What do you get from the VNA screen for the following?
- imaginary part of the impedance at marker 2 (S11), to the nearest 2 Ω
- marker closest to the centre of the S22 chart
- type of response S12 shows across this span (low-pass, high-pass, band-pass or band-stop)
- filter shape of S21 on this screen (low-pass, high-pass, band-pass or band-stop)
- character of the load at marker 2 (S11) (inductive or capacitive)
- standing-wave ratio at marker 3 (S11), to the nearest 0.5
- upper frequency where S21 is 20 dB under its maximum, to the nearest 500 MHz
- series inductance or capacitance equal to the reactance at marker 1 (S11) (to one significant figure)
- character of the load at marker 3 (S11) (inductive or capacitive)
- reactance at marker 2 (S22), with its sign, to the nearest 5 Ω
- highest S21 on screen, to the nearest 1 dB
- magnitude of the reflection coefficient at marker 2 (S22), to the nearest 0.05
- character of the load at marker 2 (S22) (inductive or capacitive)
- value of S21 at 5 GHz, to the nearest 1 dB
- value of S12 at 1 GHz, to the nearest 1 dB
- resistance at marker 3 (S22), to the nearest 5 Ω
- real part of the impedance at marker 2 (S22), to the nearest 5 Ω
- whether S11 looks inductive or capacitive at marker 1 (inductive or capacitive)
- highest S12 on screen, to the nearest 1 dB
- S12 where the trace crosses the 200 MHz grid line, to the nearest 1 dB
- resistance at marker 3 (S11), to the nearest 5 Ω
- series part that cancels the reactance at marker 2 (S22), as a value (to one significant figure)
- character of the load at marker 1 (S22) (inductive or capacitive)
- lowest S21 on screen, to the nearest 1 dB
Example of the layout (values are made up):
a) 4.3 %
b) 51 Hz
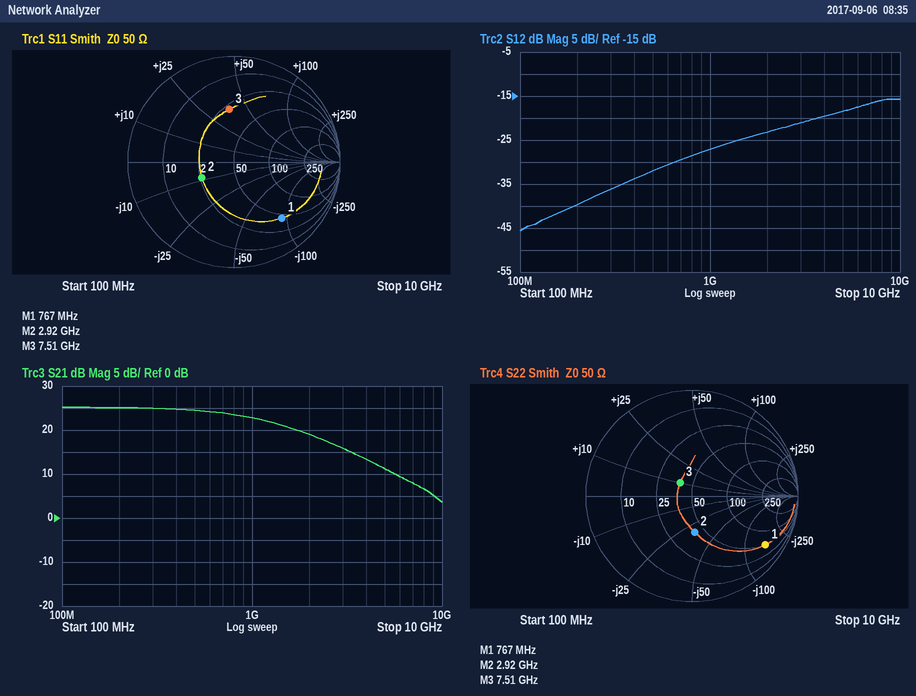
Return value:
a) -8 Ω
b) marker 3
c) high-pass
d) low-pass
e) capacitive
f) 3.0
g) 9.0 GHz
h) 2 pF
i) inductive
j) -30 Ω
k) 25 dB
l) 0.35
m) capacitive
n) 11 dB
o) -27 dB
p) 40 Ω
q) 40 Ω
r) capacitive
s) -16 dB
t) -40 dB
u) 30 Ω
v) 2 nH
w) capacitive
x) 4 dB
